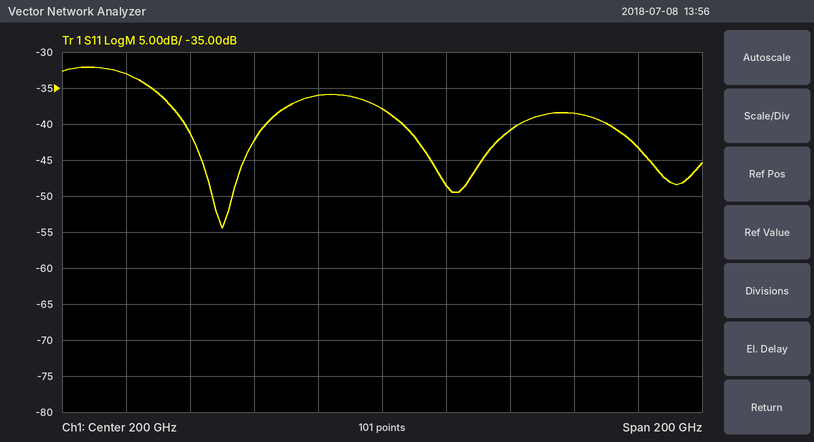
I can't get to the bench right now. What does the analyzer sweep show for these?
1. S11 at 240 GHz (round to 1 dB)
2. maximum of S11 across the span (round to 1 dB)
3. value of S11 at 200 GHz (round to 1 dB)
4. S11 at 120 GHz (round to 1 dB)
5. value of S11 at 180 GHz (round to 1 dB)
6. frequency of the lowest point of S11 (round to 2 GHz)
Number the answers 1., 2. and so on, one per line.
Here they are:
1. -41 dB
2. -32 dB
3. -38 dB
4. -33 dB
5. -36 dB
6. 150 GHz
